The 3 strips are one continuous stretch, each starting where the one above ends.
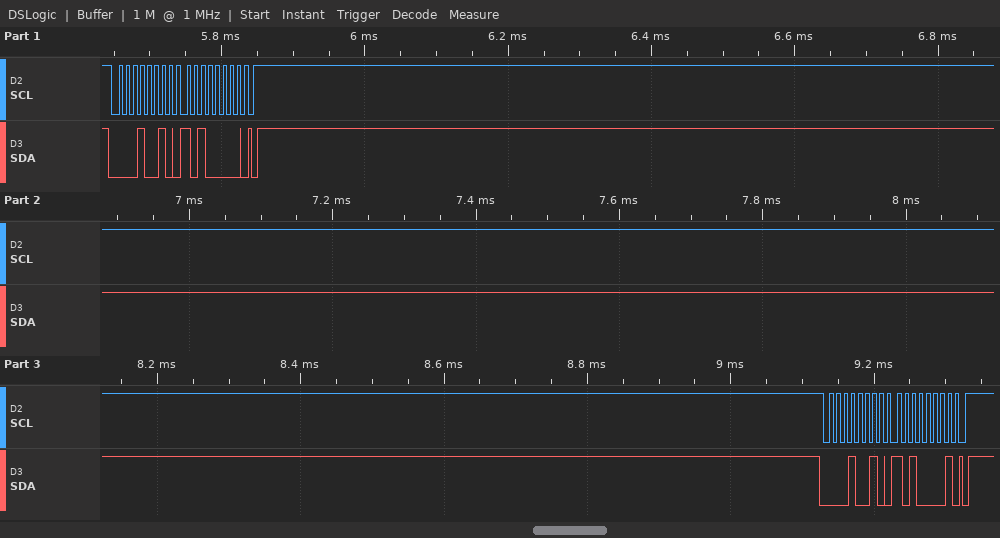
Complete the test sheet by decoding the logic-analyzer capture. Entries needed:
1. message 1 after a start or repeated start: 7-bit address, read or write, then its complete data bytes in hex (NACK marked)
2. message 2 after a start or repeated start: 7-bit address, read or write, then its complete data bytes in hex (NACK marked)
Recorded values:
0x09 write: A0
0x09 write: A1
